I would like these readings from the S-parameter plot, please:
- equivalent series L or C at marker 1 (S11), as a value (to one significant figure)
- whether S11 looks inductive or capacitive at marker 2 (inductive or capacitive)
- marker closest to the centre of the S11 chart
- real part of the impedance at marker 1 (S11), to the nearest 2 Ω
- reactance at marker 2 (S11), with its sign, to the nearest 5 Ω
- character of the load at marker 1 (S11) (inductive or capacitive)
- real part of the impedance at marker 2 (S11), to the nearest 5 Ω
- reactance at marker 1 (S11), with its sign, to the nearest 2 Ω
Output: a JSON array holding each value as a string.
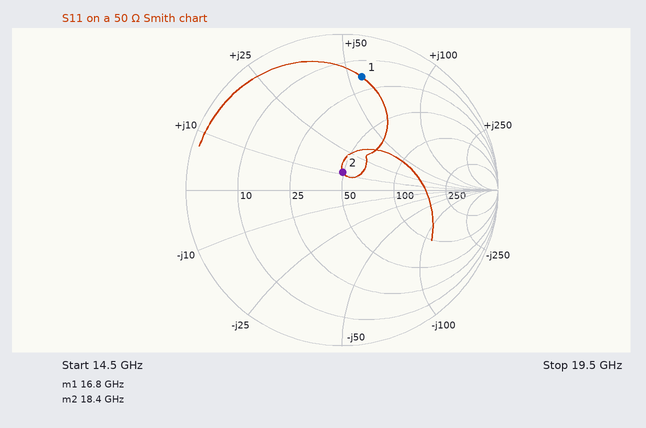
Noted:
["500 pH", "inductive", "marker 2", "18 Ω", "+10 Ω", "inductive", "50 Ω", "+56 Ω"]
